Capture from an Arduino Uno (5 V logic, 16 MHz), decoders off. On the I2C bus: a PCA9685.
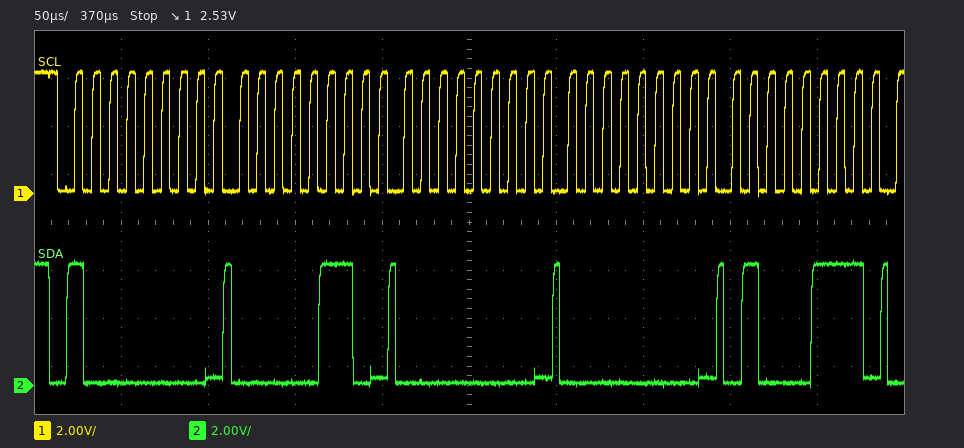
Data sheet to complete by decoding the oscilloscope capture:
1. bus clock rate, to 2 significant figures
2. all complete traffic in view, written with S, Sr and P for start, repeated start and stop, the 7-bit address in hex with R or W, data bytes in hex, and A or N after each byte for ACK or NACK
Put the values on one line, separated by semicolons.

100 kHz; S 40W A 06 A 00 A 00 A 47 A
